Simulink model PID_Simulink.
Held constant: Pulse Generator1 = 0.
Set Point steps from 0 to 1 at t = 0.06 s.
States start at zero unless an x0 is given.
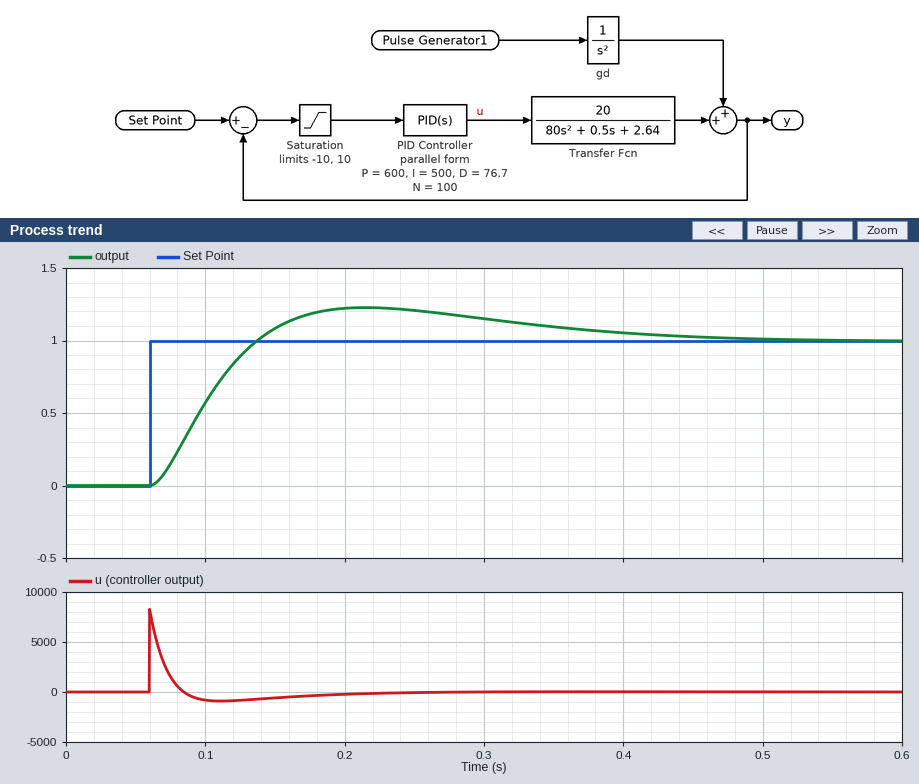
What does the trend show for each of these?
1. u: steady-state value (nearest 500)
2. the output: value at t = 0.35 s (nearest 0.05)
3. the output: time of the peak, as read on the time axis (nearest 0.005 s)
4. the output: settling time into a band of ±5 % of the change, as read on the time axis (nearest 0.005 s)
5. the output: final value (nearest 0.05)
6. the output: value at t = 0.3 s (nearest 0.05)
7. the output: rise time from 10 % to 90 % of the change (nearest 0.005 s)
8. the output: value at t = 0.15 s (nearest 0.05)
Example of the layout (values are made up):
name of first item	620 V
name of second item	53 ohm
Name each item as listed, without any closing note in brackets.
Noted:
u: steady-state value	0
the output: value at t = 0.35 s	1.10
the output: time of the peak, as read on the time axis	0.215 s
the output: settling time into a band of ±5 % of the change, as read on the time axis	0.405 s
the output: final value	1.00
the output: value at t = 0.3 s	1.15
the output: rise time from 10 % to 90 % of the change	0.055 s
the output: value at t = 0.15 s	1.10
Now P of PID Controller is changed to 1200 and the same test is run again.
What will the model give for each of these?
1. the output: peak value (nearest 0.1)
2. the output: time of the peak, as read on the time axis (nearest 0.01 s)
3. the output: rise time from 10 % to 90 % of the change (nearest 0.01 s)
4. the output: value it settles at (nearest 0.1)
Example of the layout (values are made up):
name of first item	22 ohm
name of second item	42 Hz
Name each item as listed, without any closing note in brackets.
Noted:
the output: peak value	1.3
the output: time of the peak, as read on the time axis	0.18 s
the output: rise time from 10 % to 90 % of the change	0.04 s
the output: value it settles at	1.0
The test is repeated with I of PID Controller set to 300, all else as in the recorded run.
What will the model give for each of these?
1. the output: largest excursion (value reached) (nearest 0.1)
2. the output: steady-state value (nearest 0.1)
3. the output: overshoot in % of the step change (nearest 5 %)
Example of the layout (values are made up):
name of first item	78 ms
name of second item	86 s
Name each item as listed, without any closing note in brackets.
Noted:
the output: largest excursion (value reached)	1.2
the output: steady-state value	1.0
the output: overshoot in % of the step change	20 %
